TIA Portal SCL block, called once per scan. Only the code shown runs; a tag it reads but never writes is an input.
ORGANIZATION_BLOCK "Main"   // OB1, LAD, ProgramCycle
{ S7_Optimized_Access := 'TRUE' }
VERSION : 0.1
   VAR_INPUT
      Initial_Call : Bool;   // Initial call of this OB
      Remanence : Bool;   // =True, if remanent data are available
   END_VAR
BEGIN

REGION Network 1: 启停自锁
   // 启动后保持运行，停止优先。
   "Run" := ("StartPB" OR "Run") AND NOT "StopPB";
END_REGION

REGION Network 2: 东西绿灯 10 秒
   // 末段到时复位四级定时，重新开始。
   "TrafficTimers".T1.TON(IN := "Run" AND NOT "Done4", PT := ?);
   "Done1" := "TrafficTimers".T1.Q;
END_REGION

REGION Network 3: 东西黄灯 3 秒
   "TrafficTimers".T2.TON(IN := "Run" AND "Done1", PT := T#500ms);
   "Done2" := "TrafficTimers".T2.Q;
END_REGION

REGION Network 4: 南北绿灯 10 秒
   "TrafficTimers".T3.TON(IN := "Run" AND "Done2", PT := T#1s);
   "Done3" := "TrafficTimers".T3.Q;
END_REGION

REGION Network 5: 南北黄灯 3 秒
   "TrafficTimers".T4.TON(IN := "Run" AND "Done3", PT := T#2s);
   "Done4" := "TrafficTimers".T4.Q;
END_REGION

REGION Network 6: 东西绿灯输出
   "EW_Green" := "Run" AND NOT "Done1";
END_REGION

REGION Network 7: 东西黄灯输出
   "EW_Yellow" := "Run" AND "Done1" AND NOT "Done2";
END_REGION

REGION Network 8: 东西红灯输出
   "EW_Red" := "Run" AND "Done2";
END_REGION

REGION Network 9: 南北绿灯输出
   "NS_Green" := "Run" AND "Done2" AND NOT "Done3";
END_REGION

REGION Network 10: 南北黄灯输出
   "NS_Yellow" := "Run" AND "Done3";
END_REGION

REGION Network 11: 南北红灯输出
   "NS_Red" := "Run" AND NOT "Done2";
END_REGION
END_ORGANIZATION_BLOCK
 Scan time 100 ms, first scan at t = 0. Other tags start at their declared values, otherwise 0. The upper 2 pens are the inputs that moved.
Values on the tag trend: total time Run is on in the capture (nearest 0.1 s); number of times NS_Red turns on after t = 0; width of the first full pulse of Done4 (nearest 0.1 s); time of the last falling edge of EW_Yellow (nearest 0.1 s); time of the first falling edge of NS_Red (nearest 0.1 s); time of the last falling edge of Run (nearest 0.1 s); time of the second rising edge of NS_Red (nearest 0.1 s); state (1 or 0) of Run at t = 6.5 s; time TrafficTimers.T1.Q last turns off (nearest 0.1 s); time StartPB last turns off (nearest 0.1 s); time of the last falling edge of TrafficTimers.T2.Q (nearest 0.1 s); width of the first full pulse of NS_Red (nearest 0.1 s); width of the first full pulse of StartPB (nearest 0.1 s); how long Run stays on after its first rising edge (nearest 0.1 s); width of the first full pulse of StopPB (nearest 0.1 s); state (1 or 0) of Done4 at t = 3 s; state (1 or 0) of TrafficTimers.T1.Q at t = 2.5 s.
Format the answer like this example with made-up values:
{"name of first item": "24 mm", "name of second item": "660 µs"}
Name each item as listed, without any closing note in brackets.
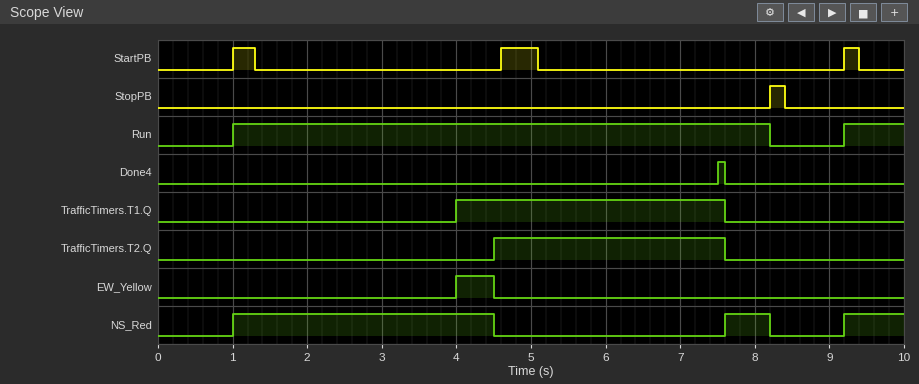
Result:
{"total time Run is on in the capture": "8.0 s", "number of times NS_Red turns on after t = 0": "3", "width of the first full pulse of Done4": "0.1 s", "time of the last falling edge of EW_Yellow": "4.5 s", "time of the first falling edge of NS_Red": "4.5 s", "time of the last falling edge of Run": "8.2 s", "time of the second rising edge of NS_Red": "7.6 s", "state (1 or 0) of Run at t = 6.5 s": "1", "time TrafficTimers.T1.Q last turns off": "7.6 s", "time StartPB last turns off": "9.4 s", "time of the last falling edge of TrafficTimers.T2.Q": "7.6 s", "width of the first full pulse of NS_Red": "3.5 s", "width of the first full pulse of StartPB": "0.3 s", "how long Run stays on after its first rising edge": "7.2 s", "width of the first full pulse of StopPB": "0.2 s", "state (1 or 0) of Done4 at t = 3 s": "0", "state (1 or 0) of TrafficTimers.T1.Q at t = 2.5 s": "0"}
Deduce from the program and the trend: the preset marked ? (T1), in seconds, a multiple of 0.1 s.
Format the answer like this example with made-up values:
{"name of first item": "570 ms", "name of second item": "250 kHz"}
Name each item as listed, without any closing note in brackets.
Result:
{"the preset marked ? (T1), in seconds, a multiple of 0.1 s": "3.0 s"}
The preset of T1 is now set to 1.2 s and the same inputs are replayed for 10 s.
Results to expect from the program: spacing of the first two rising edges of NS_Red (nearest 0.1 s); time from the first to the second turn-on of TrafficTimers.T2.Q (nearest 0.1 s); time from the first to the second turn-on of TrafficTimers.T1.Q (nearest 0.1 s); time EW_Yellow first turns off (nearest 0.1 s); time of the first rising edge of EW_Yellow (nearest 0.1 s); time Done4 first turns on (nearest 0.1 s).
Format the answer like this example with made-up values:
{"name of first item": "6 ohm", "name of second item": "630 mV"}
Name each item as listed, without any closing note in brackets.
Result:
{"spacing of the first two rising edges of NS_Red": "4.8 s", "time from the first to the second turn-on of TrafficTimers.T2.Q": "4.9 s", "time from the first to the second turn-on of TrafficTimers.T1.Q": "4.9 s", "time EW_Yellow first turns off": "2.7 s", "time of the first rising edge of EW_Yellow": "2.2 s", "time Done4 first turns on": "5.7 s"}
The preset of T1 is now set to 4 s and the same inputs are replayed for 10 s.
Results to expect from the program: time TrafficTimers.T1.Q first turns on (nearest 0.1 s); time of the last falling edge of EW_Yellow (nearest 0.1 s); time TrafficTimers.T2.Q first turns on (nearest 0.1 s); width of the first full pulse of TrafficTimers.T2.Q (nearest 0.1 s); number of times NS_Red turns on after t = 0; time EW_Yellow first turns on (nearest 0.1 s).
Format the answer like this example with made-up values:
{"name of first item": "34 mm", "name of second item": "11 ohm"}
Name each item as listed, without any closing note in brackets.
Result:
{"time TrafficTimers.T1.Q first turns on": "5.0 s", "time of the last falling edge of EW_Yellow": "5.5 s", "time TrafficTimers.T2.Q first turns on": "5.5 s", "width of the first full pulse of TrafficTimers.T2.Q": "2.7 s", "number of times NS_Red turns on after t = 0": "2", "time EW_Yellow first turns on": "5.0 s"}
